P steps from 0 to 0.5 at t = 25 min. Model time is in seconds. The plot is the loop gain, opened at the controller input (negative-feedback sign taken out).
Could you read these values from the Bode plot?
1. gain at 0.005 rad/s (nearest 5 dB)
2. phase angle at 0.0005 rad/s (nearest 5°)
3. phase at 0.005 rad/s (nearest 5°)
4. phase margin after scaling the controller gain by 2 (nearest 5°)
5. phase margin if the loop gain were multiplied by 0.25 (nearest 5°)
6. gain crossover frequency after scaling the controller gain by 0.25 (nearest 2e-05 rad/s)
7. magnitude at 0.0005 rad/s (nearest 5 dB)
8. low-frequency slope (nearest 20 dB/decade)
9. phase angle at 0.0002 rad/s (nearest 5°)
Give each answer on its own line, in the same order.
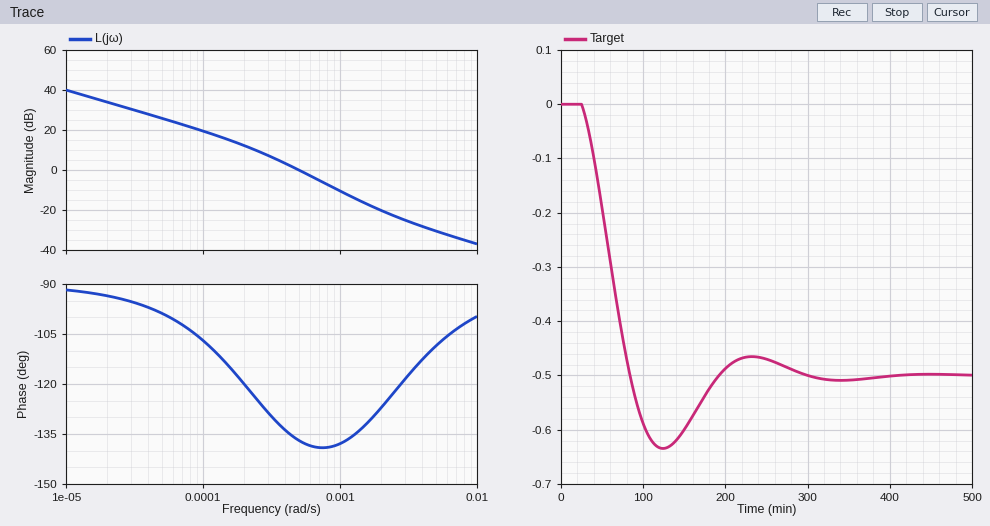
-30 dB
-135°
-110°
40°
60°
0.00020 rad/s
0 dB
-20 dB/decade
-120°
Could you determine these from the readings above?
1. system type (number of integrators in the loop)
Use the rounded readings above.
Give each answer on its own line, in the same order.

1
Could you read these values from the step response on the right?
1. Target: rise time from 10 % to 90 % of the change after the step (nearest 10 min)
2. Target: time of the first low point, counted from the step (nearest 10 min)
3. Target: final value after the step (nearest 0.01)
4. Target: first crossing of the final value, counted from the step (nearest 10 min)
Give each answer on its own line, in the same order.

40 min
100 min
-0.50
60 min
